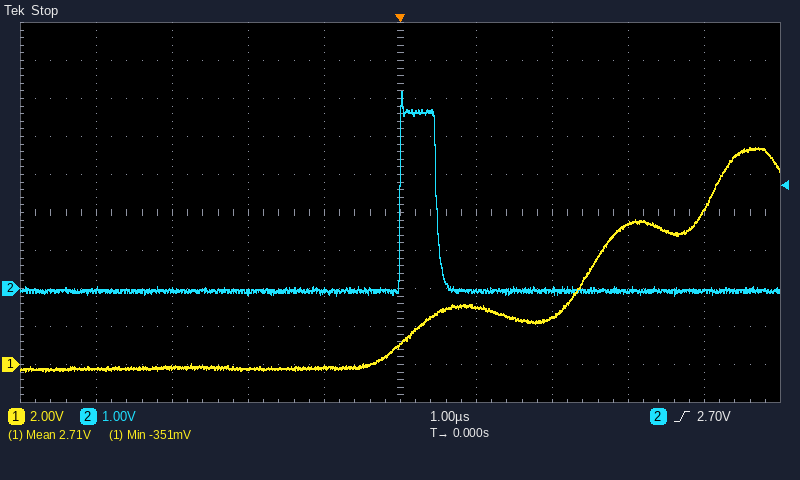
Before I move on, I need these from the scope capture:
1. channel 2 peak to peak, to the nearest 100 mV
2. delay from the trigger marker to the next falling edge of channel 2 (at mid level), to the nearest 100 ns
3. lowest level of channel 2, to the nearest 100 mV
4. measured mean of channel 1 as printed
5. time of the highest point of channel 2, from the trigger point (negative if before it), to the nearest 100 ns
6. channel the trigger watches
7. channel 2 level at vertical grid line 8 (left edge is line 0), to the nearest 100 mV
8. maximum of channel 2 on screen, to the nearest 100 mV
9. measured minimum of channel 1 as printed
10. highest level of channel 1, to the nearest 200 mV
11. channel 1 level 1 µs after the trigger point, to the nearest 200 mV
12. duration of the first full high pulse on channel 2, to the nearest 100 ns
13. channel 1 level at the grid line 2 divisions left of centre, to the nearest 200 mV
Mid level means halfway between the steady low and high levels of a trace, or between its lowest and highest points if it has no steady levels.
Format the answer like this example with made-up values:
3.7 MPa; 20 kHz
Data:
5.4 V; 500 ns; -200 mV; 2.71 V; 0.0 µs; channel 2; -100 mV; 5.2 V; -351 mV; 11.4 V; 3.0 V; 500 ns; -200 mV
